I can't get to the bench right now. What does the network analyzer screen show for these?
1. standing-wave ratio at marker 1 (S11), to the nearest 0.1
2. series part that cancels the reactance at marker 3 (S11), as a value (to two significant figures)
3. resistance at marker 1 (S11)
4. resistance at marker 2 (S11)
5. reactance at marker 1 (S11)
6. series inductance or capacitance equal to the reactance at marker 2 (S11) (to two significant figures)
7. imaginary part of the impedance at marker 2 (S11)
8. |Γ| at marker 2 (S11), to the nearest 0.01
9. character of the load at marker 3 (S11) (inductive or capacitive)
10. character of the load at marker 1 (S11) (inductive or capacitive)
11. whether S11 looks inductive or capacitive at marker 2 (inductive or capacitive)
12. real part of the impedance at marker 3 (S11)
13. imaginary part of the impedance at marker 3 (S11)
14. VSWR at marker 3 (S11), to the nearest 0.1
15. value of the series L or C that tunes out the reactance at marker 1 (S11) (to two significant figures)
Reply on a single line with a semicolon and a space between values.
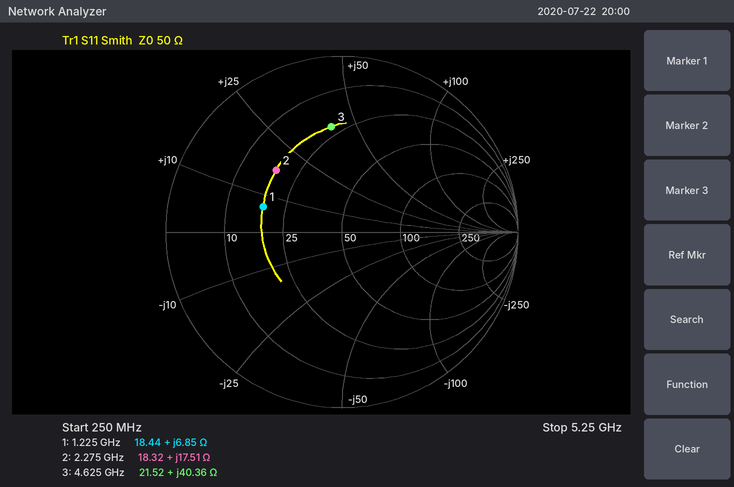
2.8; 850 fF; 18.44 Ω; 18.32 Ω; +6.85 Ω; 1.2 nH; +17.51 Ω; 0.51; inductive; inductive; inductive; 21.52 Ω; +40.36 Ω; 4.0; 19 pF
